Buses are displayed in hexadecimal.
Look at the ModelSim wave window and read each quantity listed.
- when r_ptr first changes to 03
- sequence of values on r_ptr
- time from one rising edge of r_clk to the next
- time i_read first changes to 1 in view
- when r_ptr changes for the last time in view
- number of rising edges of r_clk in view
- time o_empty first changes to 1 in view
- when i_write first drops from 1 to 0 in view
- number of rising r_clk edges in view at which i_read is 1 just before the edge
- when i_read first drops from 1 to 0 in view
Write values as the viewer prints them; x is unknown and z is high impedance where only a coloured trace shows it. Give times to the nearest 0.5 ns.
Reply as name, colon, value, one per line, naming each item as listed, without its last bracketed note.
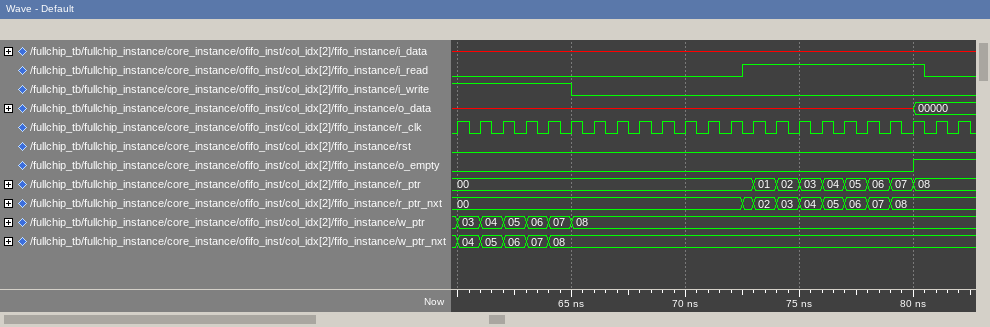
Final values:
when r_ptr first changes to 03: 75 ns
sequence of values on r_ptr: 00, 01, 02, 03, 04, 05, 06, 07, 08
time from one rising edge of r_clk to the next: 1 ns
time i_read first changes to 1 in view: 72.5 ns
when r_ptr changes for the last time in view: 80 ns
number of rising edges of r_clk in view: 23
time o_empty first changes to 1 in view: 80 ns
when i_write first drops from 1 to 0 in view: 65 ns
number of rising r_clk edges in view at which i_read is 1 just before the edge: 8
when i_read first drops from 1 to 0 in view: 80.5 ns
